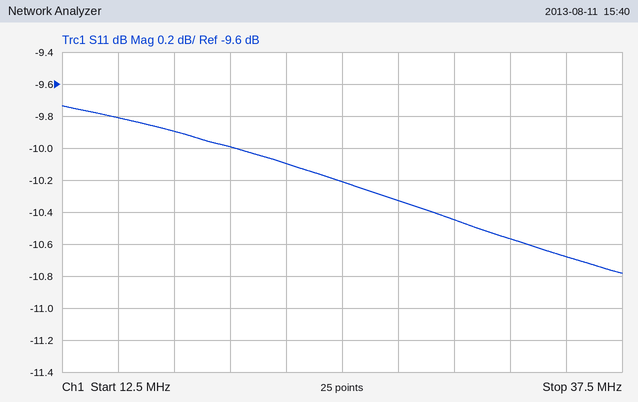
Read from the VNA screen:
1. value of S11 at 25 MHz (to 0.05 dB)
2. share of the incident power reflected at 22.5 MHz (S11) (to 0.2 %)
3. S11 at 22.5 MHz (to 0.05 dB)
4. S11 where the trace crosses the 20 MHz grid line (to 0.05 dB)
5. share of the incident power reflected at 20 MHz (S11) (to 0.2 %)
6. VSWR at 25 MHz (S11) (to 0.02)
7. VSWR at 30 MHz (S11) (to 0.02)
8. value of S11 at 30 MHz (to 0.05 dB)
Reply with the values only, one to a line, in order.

-10.20 dB
9.8 %
-10.10 dB
-10.00 dB
10.0 %
1.90
1.86
-10.45 dB
